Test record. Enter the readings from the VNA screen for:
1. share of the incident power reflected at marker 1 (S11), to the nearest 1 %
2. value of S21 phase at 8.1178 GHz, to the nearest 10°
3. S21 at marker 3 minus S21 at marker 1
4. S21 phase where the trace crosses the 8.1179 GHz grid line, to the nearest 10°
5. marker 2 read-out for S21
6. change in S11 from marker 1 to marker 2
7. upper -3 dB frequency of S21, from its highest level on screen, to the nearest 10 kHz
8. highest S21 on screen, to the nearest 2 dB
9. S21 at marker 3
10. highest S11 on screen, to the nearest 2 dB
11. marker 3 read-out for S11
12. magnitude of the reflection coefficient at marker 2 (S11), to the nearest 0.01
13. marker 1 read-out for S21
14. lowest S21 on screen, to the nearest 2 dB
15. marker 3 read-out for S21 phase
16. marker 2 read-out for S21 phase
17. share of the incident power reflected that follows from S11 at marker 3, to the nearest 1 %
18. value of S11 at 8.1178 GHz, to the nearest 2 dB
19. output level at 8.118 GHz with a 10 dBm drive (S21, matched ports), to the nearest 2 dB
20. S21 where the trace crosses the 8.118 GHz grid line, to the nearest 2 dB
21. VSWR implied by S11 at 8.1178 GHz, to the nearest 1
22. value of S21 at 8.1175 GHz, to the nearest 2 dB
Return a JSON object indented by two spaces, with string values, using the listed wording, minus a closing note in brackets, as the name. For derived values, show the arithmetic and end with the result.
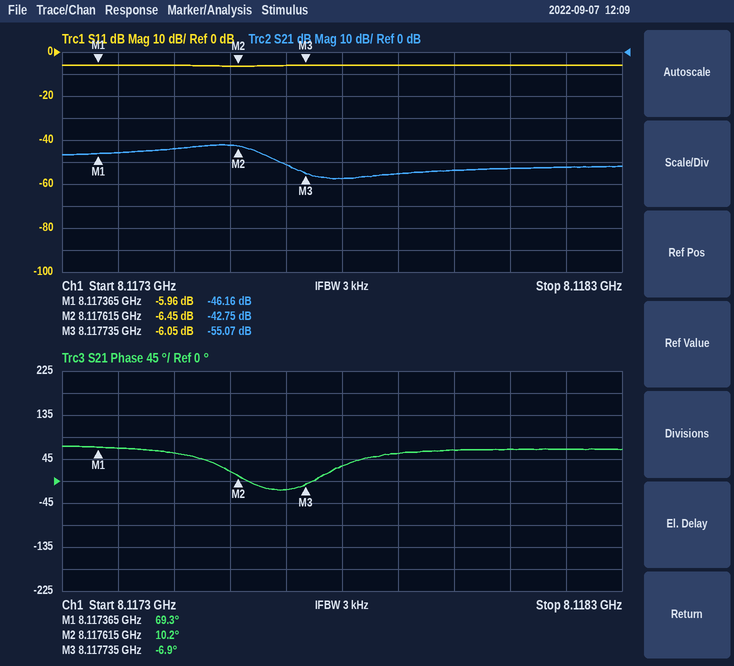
{
  "share of the incident power reflected at marker 1 (S11), to the nearest 1 %": "10^(-5.96/10) ≈ 25 %",
  "value of S21 phase at 8.1178 GHz, to the nearest 10°": "30°",
  "S21 at marker 3 minus S21 at marker 1": "-55.07 − (-46.16) = -8.91 dB",
  "S21 phase where the trace crosses the 8.1179 GHz grid line, to the nearest 10°": "60°",
  "marker 2 read-out for S21": "-42.75 dB",
  "change in S11 from marker 1 to marker 2": "-6.45 − (-5.96) = -0.49 dB",
  "upper -3 dB frequency of S21, from its highest level on screen, to the nearest 10 kHz": "8.11765 GHz",
  "highest S21 on screen, to the nearest 2 dB": "-42 dB",
  "S21 at marker 3": "-55.07 dB",
  "highest S11 on screen, to the nearest 2 dB": "-6 dB",
  "marker 3 read-out for S11": "-6.05 dB",
  "magnitude of the reflection coefficient at marker 2 (S11), to the nearest 0.01": "10^(-6.45/20) ≈ 0.48",
  "marker 1 read-out for S21": "-46.16 dB",
  "lowest S21 on screen, to the nearest 2 dB": "-58 dB",
  "marker 3 read-out for S21 phase": "-6.9°",
  "marker 2 read-out for S21 phase": "10.2°",
  "share of the incident power reflected that follows from S11 at marker 3, to the nearest 1 %": "10^(-6.05/10) ≈ 25 %",
  "value of S11 at 8.1178 GHz, to the nearest 2 dB": "-6 dB",
  "output level at 8.118 GHz with a 10 dBm drive (S21, matched ports), to the nearest 2 dB": "10 dBm + (-54 dB) = -44 dBm",
  "S21 where the trace crosses the 8.118 GHz grid line, to the nearest 2 dB": "-54 dB",
  "VSWR implied by S11 at 8.1178 GHz, to the nearest 1": "|Γ| = 10^(-6/20) = 0.5012; VSWR = (1 + 0.5012)/(1 − 0.5012) ≈ 3",
  "value of S21 at 8.1175 GHz, to the nearest 2 dB": "-44 dB"
}
